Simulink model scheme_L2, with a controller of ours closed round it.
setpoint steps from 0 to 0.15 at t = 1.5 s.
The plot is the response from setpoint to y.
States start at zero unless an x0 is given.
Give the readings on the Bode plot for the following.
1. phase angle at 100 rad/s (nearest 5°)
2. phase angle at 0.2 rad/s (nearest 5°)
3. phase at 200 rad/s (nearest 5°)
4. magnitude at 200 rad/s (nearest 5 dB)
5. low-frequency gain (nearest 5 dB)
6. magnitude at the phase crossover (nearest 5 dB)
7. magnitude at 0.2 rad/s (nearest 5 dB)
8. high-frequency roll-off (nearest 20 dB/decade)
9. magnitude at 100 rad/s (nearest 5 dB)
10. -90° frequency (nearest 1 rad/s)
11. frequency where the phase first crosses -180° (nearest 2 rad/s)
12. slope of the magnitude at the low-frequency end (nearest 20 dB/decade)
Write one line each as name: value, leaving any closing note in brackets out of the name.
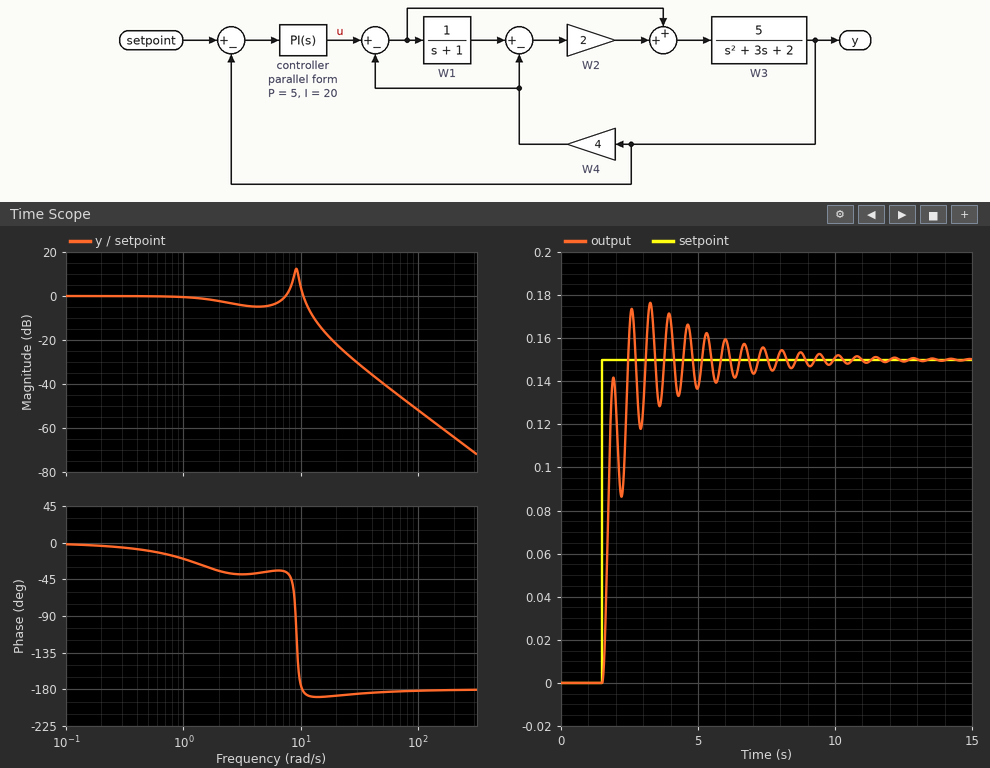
phase angle at 100 rad/s: -180°
phase angle at 0.2 rad/s: -5°
phase at 200 rad/s: -180°
magnitude at 200 rad/s: -65 dB
low-frequency gain: 0 dB
magnitude at the phase crossover: 0 dB
magnitude at 0.2 rad/s: 0 dB
high-frequency roll-off: -40 dB/decade
magnitude at 100 rad/s: -50 dB
-90° frequency: 9 rad/s
frequency where the phase first crosses -180°: 10 rad/s
slope of the magnitude at the low-frequency end: 0 dB/decade
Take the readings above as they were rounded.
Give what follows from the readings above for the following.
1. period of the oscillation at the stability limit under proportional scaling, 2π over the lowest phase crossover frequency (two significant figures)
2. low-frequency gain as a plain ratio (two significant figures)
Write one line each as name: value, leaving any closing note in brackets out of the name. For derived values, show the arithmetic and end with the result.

period of the oscillation at the stability limit under proportional scaling, 2π over the lowest phase crossover frequency: 2π / 10 = 0.63 s
low-frequency gain as a plain ratio: 10^(0 / 20) = 1.0
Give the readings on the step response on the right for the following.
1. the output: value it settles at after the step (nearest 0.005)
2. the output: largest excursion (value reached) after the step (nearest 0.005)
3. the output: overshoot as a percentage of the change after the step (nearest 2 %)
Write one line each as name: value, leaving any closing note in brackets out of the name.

the output: value it settles at after the step: 0.150
the output: largest excursion (value reached) after the step: 0.175
the output: overshoot as a percentage of the change after the step: 18 %
